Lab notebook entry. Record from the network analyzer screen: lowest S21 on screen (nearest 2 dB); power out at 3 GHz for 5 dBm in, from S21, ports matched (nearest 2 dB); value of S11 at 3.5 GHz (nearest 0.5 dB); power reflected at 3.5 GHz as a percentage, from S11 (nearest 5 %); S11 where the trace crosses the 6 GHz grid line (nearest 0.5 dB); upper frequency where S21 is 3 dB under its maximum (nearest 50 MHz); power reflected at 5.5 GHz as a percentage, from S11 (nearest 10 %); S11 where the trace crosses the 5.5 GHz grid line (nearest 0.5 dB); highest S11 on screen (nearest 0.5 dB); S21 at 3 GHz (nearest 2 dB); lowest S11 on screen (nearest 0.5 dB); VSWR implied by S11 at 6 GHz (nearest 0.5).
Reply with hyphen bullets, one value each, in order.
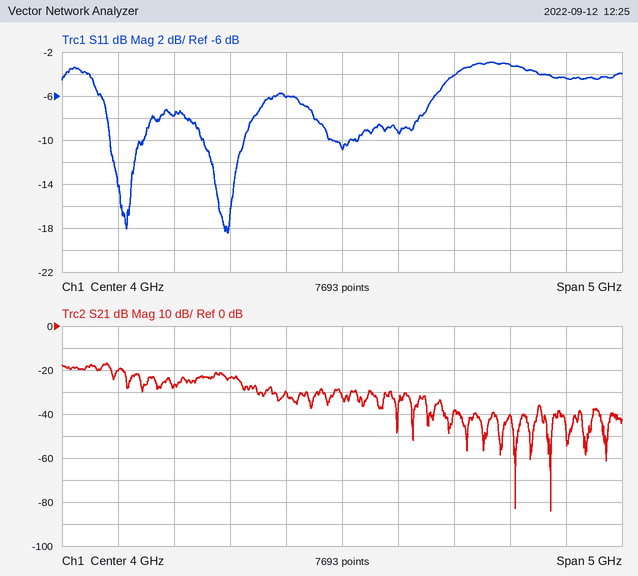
- -84 dB
- -18 dBm
- -6.0 dB
- 25 %
- -4.5 dB
- 1.95 GHz
- 50 %
- -3.0 dB
- -3.0 dB
- -24 dB
- -18.5 dB
- 4.0
